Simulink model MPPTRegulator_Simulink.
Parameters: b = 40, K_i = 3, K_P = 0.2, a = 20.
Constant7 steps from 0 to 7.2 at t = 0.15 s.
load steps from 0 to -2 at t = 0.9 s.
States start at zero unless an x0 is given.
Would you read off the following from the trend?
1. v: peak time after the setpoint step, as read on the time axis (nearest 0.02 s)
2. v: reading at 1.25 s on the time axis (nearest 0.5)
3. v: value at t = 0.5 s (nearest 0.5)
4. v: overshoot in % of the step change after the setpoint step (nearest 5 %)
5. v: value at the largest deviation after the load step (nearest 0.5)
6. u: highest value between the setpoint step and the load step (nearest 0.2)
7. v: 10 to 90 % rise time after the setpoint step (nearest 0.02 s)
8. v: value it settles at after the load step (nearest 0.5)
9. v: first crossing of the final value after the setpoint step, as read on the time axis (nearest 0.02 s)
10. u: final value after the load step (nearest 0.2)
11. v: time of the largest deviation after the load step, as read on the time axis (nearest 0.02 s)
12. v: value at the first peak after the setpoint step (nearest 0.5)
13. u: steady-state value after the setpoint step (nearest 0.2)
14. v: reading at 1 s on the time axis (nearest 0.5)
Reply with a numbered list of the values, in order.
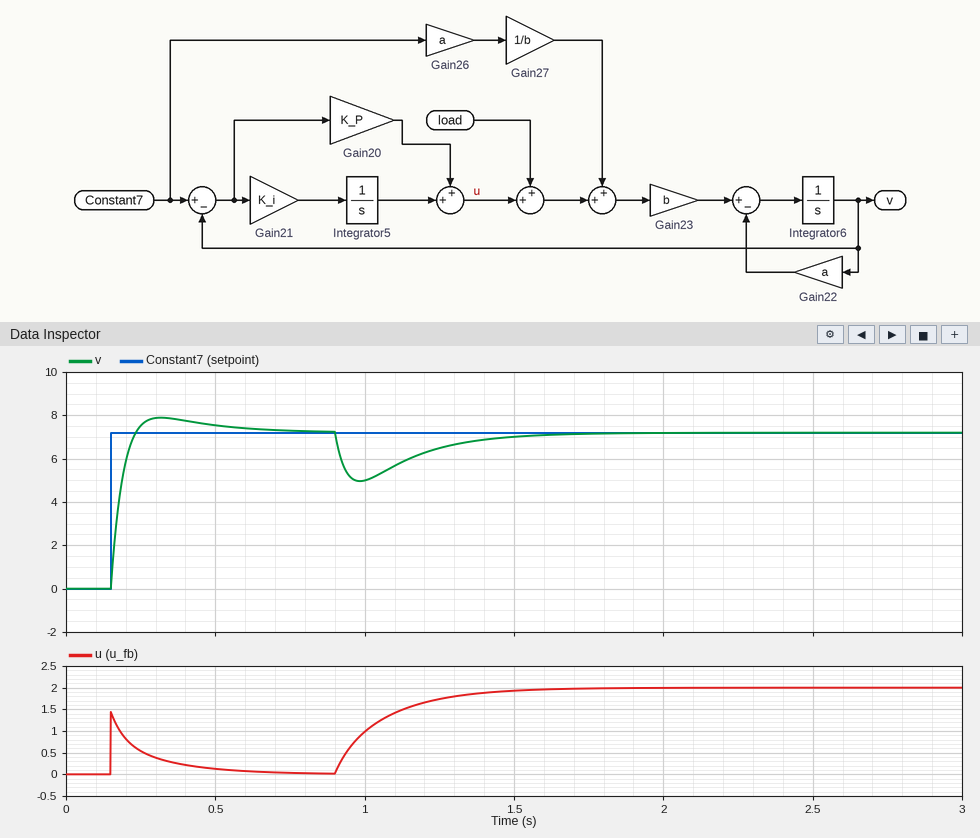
1. 0.32 s
2. 6.5
3. 7.5
4. 10 %
5. 5.0
6. 1.4
7. 0.06 s
8. 7.0
9. 0.24 s
10. 2.0
11. 0.98 s
12. 8.0
13. 0.0
14. 5.0
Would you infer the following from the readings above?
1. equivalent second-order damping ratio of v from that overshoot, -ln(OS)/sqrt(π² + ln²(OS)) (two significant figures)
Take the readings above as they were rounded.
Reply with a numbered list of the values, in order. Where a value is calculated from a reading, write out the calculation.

1. ln(0.1) = -2.303; 2.303 / sqrt(9.870 + 5.302) = 0.59
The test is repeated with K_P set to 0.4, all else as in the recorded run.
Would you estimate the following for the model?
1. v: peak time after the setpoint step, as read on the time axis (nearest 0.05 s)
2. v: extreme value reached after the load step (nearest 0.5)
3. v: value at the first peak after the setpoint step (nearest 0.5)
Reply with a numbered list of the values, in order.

1. 0.30 s
2. 5.5
3. 7.5
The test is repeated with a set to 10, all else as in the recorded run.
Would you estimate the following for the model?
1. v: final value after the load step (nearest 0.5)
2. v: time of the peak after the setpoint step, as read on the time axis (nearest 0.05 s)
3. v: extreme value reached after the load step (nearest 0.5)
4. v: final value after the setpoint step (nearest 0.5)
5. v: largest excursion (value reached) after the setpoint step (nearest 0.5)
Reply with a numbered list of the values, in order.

1. 7.0
2. 0.35 s
3. 4.0
4. 7.0
5. 8.5
